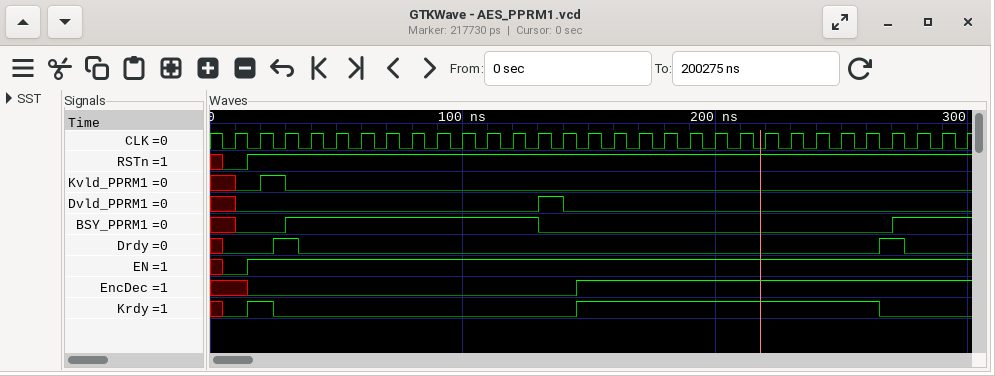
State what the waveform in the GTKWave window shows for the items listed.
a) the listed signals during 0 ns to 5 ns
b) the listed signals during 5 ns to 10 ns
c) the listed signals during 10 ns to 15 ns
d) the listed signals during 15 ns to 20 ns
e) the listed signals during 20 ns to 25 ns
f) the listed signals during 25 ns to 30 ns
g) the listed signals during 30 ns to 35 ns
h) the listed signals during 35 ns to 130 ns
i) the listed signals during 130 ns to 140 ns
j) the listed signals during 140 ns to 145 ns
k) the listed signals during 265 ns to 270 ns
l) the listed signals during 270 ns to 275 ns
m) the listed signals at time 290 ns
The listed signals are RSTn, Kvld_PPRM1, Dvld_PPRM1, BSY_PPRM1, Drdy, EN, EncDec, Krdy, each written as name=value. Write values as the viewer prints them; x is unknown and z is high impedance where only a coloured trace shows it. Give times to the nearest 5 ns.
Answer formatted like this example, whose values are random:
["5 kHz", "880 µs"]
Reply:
["RSTn=x, Kvld_PPRM1=x, Dvld_PPRM1=x, BSY_PPRM1=x, Drdy=x, EN=x, EncDec=x, Krdy=x", "RSTn=0, Kvld_PPRM1=x, Dvld_PPRM1=x, BSY_PPRM1=x, Drdy=0, EN=0, EncDec=x, Krdy=0", "RSTn=0, Kvld_PPRM1=0, Dvld_PPRM1=0, BSY_PPRM1=0, Drdy=0, EN=0, EncDec=x, Krdy=0", "RSTn=1, Kvld_PPRM1=0, Dvld_PPRM1=0, BSY_PPRM1=0, Drdy=0, EN=1, EncDec=0, Krdy=1", "RSTn=1, Kvld_PPRM1=1, Dvld_PPRM1=0, BSY_PPRM1=0, Drdy=0, EN=1, EncDec=0, Krdy=1", "RSTn=1, Kvld_PPRM1=1, Dvld_PPRM1=0, BSY_PPRM1=0, Drdy=1, EN=1, EncDec=0, Krdy=0", "RSTn=1, Kvld_PPRM1=0, Dvld_PPRM1=0, BSY_PPRM1=1, Drdy=1, EN=1, EncDec=0, Krdy=0", "RSTn=1, Kvld_PPRM1=0, Dvld_PPRM1=0, BSY_PPRM1=1, Drdy=0, EN=1, EncDec=0, Krdy=0", "RSTn=1, Kvld_PPRM1=0, Dvld_PPRM1=1, BSY_PPRM1=0, Drdy=0, EN=1, EncDec=0, Krdy=0", "RSTn=1, Kvld_PPRM1=0, Dvld_PPRM1=0, BSY_PPRM1=0, Drdy=0, EN=1, EncDec=0, Krdy=0", "RSTn=1, Kvld_PPRM1=0, Dvld_PPRM1=0, BSY_PPRM1=0, Drdy=1, EN=1, EncDec=1, Krdy=0", "RSTn=1, Kvld_PPRM1=0, Dvld_PPRM1=0, BSY_PPRM1=1, Drdy=1, EN=1, EncDec=1, Krdy=0", "RSTn=1, Kvld_PPRM1=0, Dvld_PPRM1=0, BSY_PPRM1=1, Drdy=0, EN=1, EncDec=1, Krdy=0"]
